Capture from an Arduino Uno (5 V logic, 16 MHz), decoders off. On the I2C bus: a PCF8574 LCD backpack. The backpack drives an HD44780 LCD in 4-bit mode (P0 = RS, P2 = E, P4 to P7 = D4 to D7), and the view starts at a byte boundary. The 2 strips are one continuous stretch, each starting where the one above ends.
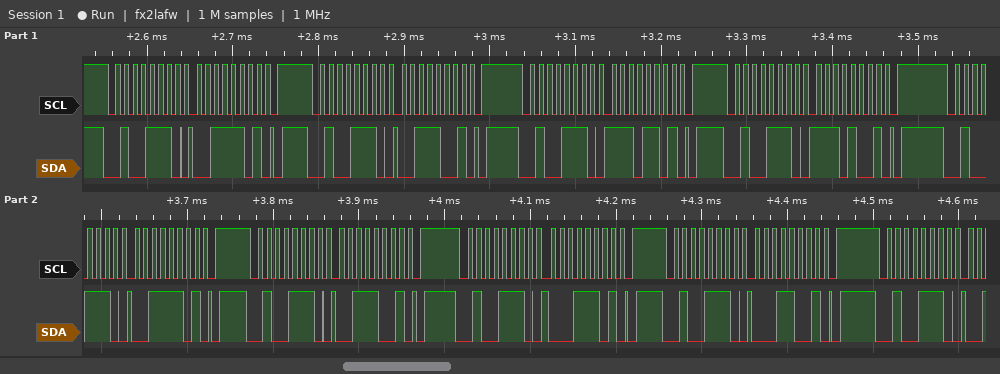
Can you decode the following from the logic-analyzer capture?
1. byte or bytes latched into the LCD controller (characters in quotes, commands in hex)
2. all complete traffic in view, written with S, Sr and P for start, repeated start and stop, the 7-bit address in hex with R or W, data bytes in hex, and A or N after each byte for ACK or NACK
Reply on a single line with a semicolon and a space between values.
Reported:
'>' '1'; S 27W A 3D A P S 27W A 39 A P S 27W A ED A P S 27W A E9 A P S 27W A 3D A P S 27W A 39 A P S 27W A 1D A P S 27W A 19 A P S 27W A
